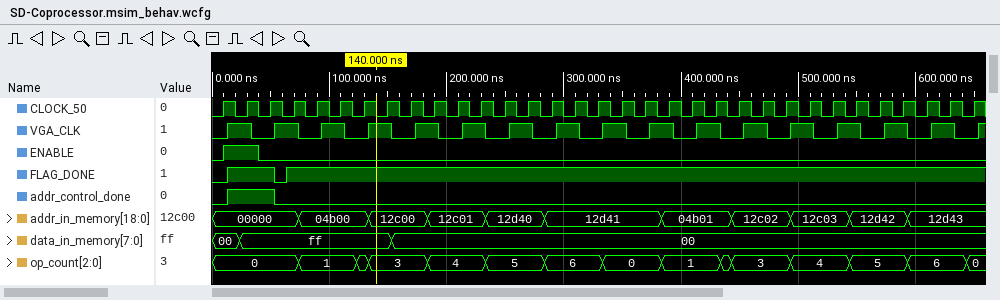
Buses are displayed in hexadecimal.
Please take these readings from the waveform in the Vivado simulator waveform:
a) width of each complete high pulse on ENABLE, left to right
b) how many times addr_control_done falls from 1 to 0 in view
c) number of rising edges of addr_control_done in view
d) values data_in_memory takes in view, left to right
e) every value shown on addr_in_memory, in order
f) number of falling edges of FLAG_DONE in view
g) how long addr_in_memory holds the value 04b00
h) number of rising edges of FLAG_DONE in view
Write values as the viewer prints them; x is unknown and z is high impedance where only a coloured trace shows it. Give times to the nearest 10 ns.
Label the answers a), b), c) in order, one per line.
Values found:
a) 30 ns
b) 1
c) 1
d) 00, ff, 00
e) 00000, 04b00, 12c00, 12c01, 12d40, 12d41, 04b01, 12c02, 12c03, 12d42, 12d43
f) 1
g) 60 ns
h) 2
